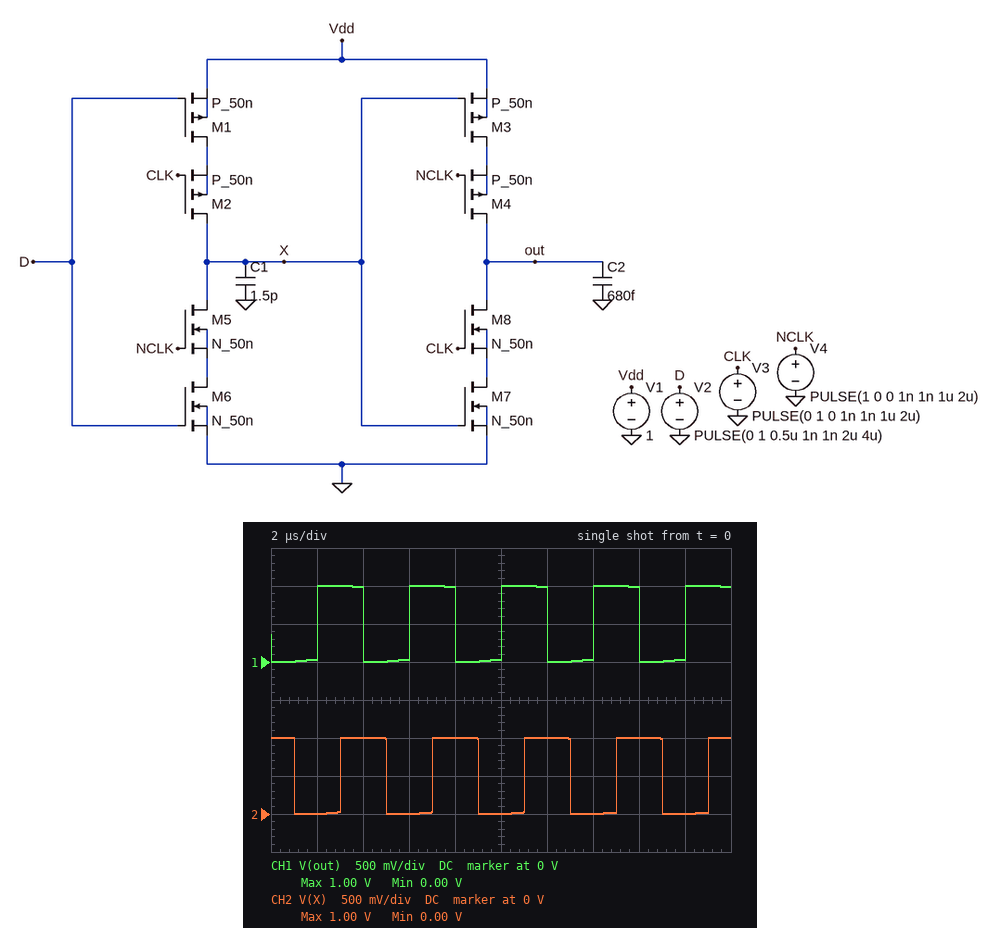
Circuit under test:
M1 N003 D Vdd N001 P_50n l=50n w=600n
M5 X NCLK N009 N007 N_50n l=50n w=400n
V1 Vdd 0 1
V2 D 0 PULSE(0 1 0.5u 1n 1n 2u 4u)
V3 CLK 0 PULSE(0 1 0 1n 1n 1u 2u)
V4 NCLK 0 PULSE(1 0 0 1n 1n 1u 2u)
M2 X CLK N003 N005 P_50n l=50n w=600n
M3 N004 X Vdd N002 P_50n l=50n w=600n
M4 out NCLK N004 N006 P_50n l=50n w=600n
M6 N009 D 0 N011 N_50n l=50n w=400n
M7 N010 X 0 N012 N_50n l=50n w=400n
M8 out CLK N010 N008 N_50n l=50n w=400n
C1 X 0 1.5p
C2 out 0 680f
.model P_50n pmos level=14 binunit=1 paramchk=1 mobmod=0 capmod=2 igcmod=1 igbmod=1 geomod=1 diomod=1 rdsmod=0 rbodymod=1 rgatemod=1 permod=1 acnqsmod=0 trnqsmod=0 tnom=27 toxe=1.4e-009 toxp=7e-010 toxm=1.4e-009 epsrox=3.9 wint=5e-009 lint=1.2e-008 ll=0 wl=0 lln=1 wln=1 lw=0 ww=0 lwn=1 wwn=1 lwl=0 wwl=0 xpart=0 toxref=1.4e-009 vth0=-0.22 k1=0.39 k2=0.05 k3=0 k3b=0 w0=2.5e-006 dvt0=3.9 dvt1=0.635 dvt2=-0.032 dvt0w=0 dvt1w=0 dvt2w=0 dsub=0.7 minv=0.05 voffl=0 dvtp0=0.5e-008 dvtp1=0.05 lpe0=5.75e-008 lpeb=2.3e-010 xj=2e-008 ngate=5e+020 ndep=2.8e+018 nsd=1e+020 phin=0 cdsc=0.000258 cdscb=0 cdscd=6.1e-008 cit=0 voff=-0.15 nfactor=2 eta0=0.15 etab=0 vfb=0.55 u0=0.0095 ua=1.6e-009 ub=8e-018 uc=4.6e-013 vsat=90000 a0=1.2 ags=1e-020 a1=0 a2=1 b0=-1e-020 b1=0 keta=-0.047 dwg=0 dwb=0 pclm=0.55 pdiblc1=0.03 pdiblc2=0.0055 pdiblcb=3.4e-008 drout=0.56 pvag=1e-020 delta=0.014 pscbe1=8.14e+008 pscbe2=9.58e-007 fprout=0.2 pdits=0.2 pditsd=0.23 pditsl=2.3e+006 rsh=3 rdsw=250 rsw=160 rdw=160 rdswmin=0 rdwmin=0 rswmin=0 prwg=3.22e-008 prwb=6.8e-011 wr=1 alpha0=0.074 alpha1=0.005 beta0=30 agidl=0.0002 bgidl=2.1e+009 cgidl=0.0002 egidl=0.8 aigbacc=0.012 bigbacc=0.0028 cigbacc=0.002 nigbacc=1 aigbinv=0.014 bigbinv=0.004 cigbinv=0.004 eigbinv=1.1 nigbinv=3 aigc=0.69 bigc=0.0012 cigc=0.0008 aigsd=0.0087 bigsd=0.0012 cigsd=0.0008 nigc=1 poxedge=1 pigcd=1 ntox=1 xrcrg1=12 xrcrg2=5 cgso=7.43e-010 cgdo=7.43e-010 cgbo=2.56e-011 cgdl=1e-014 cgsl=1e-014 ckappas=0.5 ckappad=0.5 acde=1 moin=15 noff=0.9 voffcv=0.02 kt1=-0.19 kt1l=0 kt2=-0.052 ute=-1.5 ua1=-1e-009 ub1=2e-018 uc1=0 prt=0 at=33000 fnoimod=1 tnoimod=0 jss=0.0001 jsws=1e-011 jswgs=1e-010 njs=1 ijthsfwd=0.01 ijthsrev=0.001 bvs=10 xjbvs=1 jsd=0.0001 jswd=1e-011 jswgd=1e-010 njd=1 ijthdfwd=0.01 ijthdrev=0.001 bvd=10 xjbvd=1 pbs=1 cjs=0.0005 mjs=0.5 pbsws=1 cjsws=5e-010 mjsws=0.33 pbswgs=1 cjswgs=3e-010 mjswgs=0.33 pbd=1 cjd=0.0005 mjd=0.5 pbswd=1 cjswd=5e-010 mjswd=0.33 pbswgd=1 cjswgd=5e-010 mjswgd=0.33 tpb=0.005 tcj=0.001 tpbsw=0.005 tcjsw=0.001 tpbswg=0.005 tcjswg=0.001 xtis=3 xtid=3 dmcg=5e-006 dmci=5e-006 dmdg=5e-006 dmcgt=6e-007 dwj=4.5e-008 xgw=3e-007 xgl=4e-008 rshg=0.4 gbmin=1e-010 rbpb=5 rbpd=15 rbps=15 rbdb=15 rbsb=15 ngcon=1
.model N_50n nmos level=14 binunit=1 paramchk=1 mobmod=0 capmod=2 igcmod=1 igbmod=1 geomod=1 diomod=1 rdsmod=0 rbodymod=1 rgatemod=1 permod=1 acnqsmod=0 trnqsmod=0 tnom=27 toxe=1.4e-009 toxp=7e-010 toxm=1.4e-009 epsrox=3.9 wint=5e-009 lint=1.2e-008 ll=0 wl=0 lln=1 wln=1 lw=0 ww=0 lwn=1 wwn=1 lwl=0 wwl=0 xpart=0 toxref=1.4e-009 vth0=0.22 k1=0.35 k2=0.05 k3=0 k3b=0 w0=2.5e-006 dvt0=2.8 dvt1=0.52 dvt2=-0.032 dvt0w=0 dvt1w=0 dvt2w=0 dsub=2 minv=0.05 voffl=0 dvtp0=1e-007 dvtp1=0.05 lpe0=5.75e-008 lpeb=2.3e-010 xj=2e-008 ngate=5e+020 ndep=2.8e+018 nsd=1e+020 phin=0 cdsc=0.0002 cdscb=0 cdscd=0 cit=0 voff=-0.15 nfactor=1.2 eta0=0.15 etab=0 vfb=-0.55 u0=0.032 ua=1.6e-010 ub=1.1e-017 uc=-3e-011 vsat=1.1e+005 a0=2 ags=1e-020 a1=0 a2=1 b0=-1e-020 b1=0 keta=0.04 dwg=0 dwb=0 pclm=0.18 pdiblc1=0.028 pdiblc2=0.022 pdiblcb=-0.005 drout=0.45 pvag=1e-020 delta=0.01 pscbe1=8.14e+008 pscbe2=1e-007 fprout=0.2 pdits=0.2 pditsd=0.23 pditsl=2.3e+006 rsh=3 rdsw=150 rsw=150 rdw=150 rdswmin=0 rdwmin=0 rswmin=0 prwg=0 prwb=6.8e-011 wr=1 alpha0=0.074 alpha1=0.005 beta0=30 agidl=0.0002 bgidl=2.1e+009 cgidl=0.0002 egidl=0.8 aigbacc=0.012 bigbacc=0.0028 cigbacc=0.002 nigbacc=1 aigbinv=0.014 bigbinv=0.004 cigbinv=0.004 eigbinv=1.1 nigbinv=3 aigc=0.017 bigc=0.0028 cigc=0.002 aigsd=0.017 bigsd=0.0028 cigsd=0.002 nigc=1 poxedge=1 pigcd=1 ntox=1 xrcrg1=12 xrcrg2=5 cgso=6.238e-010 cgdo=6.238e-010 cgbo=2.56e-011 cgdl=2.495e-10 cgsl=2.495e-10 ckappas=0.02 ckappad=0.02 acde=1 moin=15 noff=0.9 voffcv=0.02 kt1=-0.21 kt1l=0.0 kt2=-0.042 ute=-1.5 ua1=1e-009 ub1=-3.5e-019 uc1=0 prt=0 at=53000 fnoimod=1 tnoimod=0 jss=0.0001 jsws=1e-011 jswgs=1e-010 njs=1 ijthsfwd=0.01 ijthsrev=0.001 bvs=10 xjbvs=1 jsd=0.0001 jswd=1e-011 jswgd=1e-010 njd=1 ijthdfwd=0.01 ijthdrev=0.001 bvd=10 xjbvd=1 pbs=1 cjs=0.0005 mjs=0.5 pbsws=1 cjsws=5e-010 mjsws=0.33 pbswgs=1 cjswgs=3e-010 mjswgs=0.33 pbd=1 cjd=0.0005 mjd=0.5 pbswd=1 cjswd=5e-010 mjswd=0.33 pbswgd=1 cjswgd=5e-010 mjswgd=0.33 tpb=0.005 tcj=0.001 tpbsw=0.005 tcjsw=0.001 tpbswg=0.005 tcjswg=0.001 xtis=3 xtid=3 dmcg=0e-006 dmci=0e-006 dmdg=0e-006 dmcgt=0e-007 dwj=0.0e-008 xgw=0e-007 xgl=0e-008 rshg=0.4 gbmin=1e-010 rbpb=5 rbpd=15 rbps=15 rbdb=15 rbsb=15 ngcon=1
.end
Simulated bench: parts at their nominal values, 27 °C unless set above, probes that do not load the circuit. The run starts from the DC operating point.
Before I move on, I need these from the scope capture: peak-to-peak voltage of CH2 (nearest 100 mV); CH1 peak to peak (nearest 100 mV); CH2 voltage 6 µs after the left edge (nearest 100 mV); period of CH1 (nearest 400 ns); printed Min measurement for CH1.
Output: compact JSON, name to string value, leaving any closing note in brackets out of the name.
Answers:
{"peak-to-peak voltage of CH2": "1.0 V", "CH1 peak to peak": "1.0 V", "CH2 voltage 6 µs after the left edge": "0 V", "period of CH1": "4.0 µs", "printed Min measurement for CH1": "0.00 V"}
